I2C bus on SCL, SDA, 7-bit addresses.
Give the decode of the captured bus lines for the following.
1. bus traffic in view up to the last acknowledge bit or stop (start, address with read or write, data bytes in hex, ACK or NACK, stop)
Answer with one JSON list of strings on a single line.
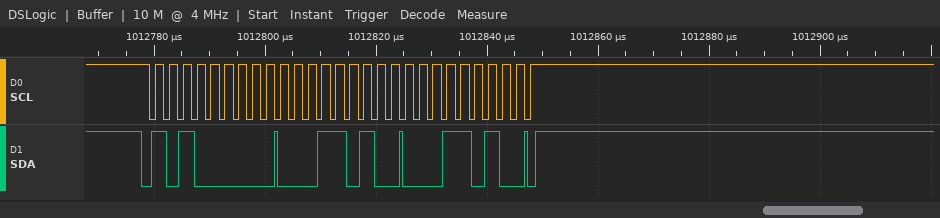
["start, address 50 write ACK, 1A ACK, 1A ACK, stop"]
